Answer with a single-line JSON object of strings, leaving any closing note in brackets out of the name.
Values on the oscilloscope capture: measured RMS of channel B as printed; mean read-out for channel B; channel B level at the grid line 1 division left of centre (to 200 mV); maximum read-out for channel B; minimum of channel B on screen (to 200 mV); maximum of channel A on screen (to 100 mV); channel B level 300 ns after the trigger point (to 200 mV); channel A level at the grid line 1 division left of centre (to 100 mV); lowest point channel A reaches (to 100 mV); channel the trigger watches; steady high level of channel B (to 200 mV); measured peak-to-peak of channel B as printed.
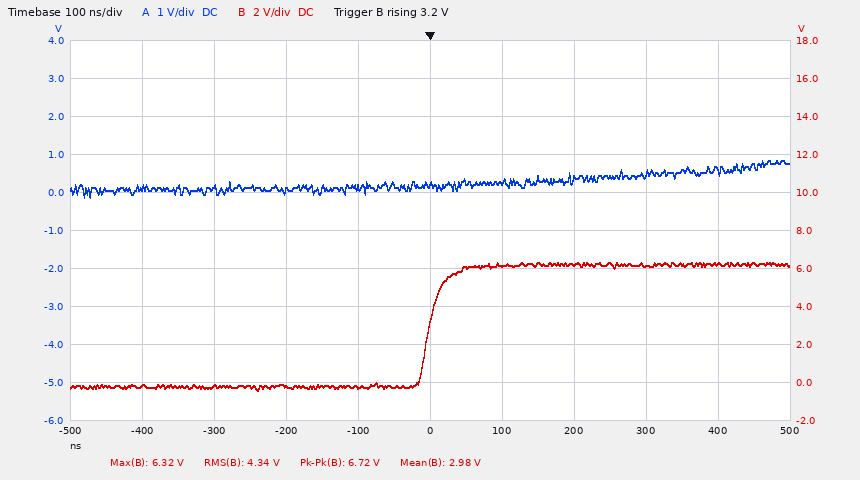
{"measured RMS of channel B as printed": "4.34 V", "mean read-out for channel B": "2.98 V", "channel B level at the grid line 1 division left of centre": "-200 mV", "maximum read-out for channel B": "6.32 V", "minimum of channel B on screen": "-400 mV", "maximum of channel A on screen": "800 mV", "channel B level 300 ns after the trigger point": "6.2 V", "channel A level at the grid line 1 division left of centre": "100 mV", "lowest point channel A reaches": "-100 mV", "channel the trigger watches": "channel B", "steady high level of channel B": "6.2 V", "measured peak-to-peak of channel B as printed": "6.72 V"}
